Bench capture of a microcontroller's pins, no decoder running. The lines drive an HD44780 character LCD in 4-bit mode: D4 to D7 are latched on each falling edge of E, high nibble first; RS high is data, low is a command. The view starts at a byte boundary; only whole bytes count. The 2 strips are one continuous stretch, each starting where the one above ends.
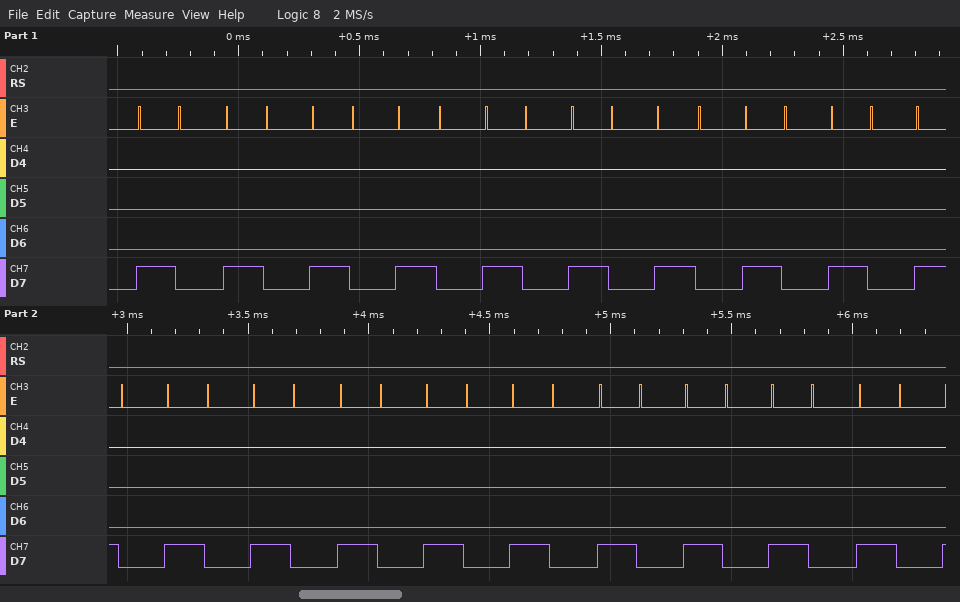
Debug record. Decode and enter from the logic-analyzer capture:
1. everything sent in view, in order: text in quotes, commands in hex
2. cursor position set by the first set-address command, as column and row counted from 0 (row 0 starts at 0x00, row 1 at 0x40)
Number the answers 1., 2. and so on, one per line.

1. 0x80 0x80 0x80 0x80 0x80 0x80 0x80 0x80 0x80 0x80 0x80 0x80 0x80 0x80 0x80 0x80 0x80 0x80 0x80
2. column 0, row 0
